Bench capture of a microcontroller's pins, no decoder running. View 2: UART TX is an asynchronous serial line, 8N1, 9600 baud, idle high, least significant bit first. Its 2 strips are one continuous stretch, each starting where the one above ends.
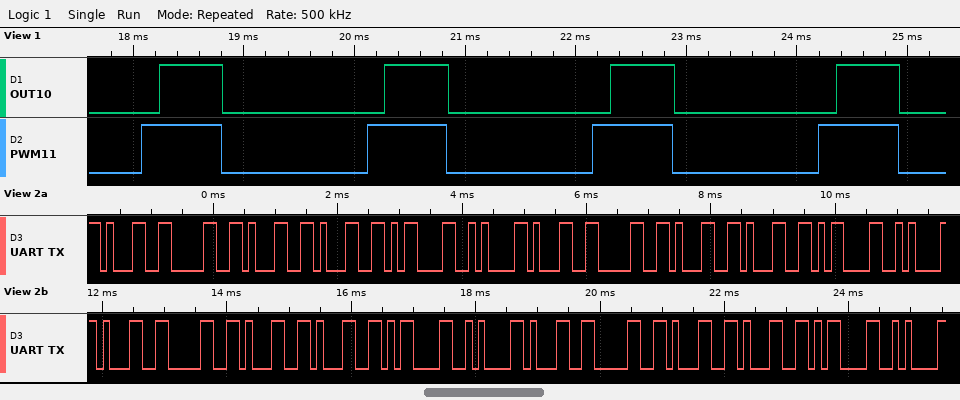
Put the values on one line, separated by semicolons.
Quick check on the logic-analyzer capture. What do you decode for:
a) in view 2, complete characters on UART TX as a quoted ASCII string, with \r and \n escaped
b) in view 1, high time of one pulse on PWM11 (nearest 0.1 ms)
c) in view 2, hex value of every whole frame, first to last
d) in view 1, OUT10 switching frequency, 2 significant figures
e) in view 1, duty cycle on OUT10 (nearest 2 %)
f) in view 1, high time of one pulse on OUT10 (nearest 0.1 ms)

"1011\r\n1011\r\n1011\r\n1011\r\n"; 0.7 ms; 0x31 0x30 0x31 0x31 0x0D 0x0A 0x31 0x30 0x31 0x31 0x0D 0x0A 0x31 0x30 0x31 0x31 0x0D 0x0A 0x31 0x30 0x31 0x31 0x0D 0x0A; 490 Hz; 28 %; 0.6 ms
